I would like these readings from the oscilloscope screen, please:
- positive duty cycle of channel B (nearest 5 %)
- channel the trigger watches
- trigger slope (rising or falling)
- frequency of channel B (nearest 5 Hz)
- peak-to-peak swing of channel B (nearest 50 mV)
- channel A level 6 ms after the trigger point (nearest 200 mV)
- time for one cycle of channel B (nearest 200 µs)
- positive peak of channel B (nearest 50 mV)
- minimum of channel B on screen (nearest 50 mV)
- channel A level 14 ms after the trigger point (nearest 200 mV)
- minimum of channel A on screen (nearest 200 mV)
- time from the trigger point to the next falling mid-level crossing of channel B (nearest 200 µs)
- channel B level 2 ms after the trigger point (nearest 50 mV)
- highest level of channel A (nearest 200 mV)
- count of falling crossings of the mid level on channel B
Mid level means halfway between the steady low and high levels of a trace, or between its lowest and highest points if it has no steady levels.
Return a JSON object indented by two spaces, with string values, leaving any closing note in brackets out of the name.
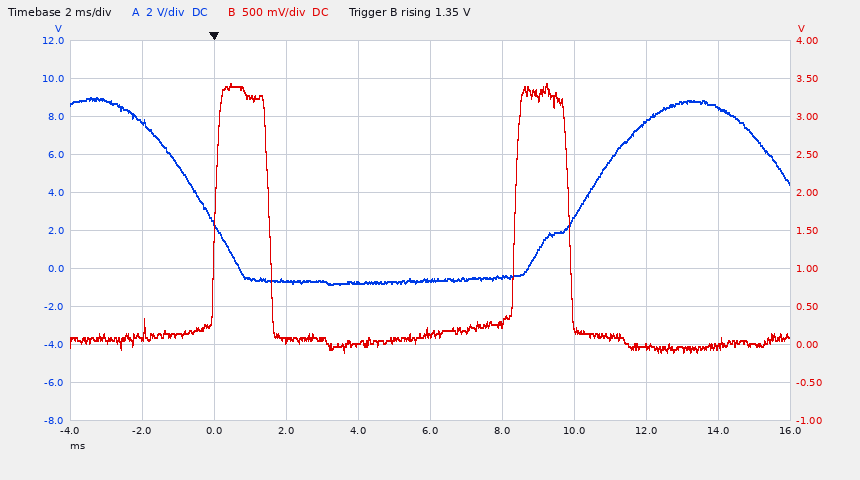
{
  "positive duty cycle of channel B": "20 %",
  "channel the trigger watches": "channel B",
  "trigger slope": "rising",
  "frequency of channel B": "120 Hz",
  "peak-to-peak swing of channel B": "3.55 V",
  "channel A level 6 ms after the trigger point": "-600 mV",
  "time for one cycle of channel B": "8.4 ms",
  "positive peak of channel B": "3.45 V",
  "minimum of channel B on screen": "-100 mV",
  "channel A level 14 ms after the trigger point": "8.4 V",
  "minimum of channel A on screen": "-800 mV",
  "time from the trigger point to the next falling mid-level crossing of channel B": "1.6 ms",
  "channel B level 2 ms after the trigger point": "50 mV",
  "highest level of channel A": "9.0 V",
  "count of falling crossings of the mid level on channel B": "2"
}
